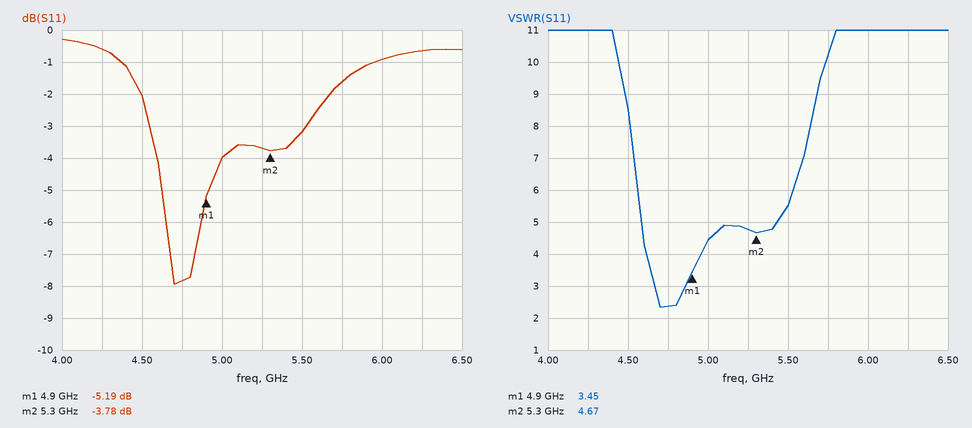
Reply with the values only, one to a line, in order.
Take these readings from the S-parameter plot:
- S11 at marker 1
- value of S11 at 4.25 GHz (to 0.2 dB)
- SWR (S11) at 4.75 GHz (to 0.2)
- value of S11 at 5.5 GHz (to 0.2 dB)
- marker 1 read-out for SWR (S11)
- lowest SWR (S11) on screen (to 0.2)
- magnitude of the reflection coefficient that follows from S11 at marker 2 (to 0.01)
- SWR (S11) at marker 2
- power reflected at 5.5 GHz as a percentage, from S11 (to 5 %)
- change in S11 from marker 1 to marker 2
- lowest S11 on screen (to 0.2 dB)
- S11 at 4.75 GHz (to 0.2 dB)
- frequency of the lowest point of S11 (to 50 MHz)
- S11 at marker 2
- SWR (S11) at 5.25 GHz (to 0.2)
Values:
-5.19 dB
-0.6 dB
2.4
-3.2 dB
3.45
2.4
0.65
4.67
50 %
1.41 dB
-8.0 dB
-7.8 dB
4.70 GHz
-3.78 dB
4.8
